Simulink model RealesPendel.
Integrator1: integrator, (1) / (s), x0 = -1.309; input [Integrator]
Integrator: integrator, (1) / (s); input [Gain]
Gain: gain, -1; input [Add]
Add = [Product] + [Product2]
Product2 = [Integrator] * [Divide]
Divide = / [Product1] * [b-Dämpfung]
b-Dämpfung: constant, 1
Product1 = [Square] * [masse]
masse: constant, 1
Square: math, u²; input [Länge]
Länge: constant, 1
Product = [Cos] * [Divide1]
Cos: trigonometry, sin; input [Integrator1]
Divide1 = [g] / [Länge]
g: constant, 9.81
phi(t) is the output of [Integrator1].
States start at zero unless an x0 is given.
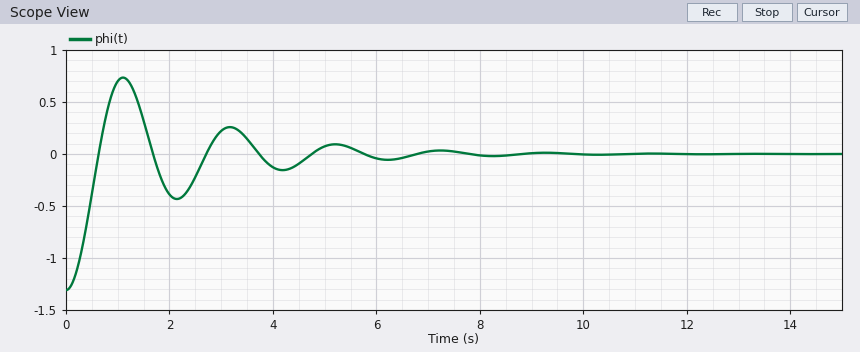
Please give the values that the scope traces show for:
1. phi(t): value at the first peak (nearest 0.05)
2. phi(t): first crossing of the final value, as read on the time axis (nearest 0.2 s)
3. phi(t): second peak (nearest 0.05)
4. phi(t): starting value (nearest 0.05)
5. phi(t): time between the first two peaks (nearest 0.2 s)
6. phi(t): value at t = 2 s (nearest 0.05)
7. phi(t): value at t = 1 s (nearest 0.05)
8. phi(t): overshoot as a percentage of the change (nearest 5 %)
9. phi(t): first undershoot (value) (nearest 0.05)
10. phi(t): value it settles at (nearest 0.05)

0.75
0.6 s
0.25
-1.30
2.0 s
-0.40
0.70
55 %
-0.45
0.00
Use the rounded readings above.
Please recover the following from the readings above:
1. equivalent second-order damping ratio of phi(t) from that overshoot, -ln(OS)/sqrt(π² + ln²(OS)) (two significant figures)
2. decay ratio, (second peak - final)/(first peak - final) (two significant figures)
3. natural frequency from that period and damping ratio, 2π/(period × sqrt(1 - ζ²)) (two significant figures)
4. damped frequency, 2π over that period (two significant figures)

0.19
0.33
3.2 rad/s
3.1 rad/s
